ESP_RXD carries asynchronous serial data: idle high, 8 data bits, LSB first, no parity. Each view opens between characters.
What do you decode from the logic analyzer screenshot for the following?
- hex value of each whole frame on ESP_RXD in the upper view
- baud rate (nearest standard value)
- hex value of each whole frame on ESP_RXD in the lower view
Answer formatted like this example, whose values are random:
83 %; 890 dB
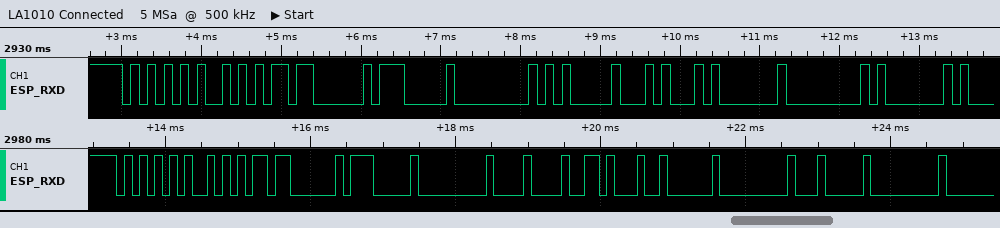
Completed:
55, AA, 03, 07, 00, 05, 14, 01, 00, 01; 9600 baud; 55, AA, 03, 07, 00, 08, 16, 02, 00, 04, 00
